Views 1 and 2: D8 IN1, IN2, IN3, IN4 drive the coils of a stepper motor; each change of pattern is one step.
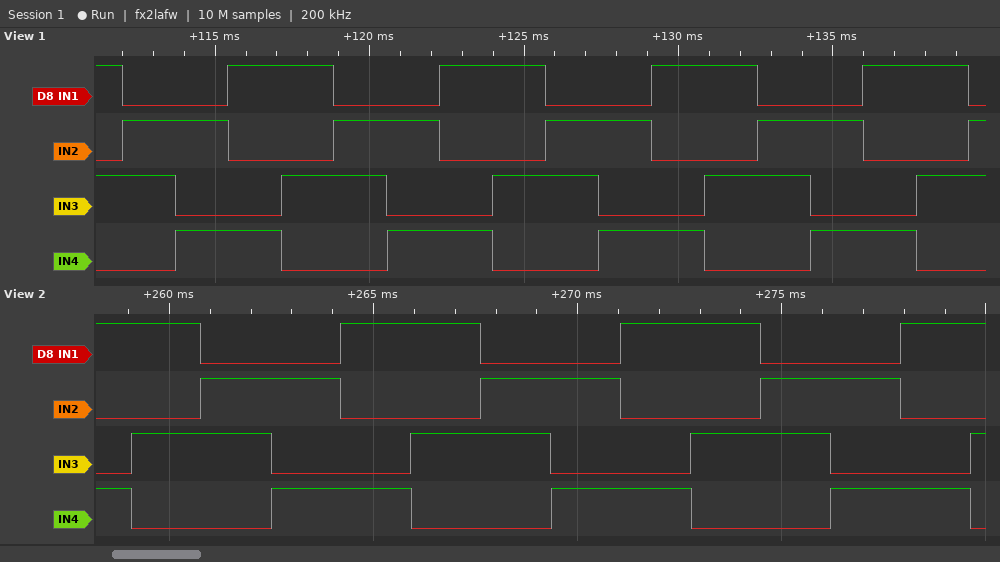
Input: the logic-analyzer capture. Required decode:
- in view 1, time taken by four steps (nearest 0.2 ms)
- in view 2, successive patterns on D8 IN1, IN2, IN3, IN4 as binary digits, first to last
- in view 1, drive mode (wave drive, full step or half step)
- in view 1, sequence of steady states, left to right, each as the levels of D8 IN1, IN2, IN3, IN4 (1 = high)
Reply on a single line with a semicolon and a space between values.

6.8 ms; 1001 1010 0110 0101 1001 1010 0110 0101 1001 1010 0110 0101 1001 1010; full step; 1010 0110 0101 1001 1010 0110 0101 1001 1010 0110 0101 1001 1010 0110 0101 1001 1010 0110
